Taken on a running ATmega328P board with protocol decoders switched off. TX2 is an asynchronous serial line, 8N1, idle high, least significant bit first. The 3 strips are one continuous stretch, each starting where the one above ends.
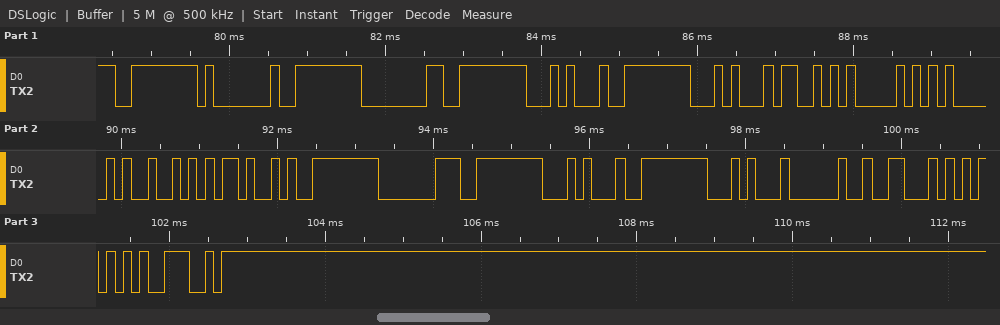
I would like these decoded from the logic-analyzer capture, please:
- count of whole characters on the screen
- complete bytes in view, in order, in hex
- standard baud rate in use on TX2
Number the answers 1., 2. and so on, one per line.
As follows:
1. 23
2. FE 01 FE 80 FE 14 FE 14 53 50 41 52 4B FE C0 FE 14 FE 14 20 46 55 4E
3. 9600 baud
